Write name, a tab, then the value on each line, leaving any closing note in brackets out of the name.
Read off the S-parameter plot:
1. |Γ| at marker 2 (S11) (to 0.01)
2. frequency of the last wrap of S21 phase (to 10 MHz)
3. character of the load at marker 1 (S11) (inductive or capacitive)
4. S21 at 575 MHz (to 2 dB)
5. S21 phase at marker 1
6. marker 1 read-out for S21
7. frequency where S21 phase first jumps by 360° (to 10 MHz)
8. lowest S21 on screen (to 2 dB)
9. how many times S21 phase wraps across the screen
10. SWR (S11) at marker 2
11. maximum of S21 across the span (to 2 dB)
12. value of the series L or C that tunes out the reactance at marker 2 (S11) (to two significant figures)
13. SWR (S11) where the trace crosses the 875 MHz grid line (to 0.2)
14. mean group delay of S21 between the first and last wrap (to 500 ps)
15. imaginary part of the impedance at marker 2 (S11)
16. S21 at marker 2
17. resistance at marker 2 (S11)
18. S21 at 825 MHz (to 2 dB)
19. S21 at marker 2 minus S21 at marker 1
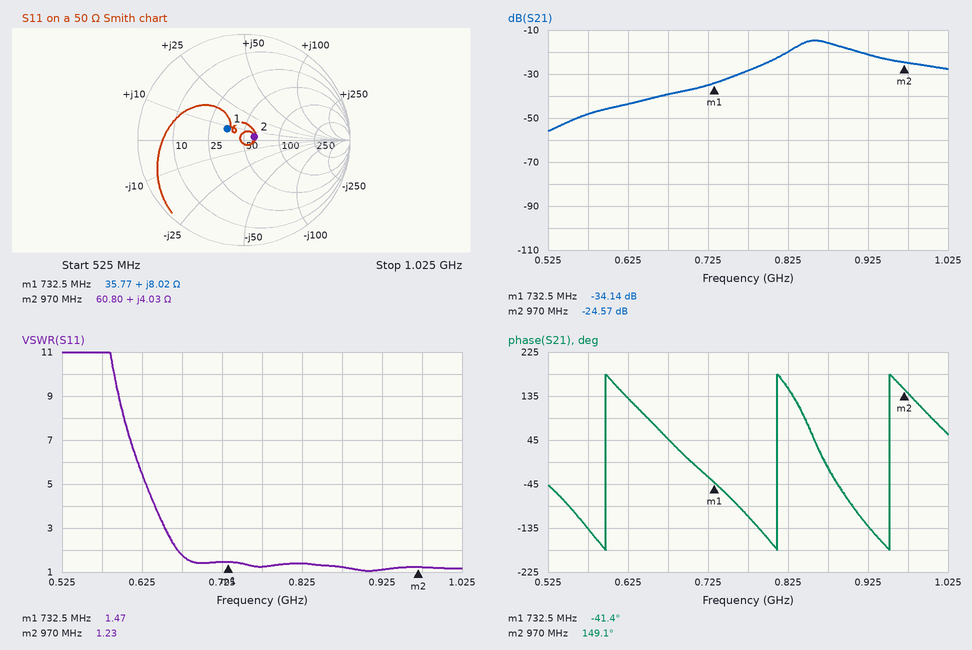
|Γ| at marker 2 (S11)	0.10
frequency of the last wrap of S21 phase	950 MHz
character of the load at marker 1 (S11)	inductive
S21 at 575 MHz	-48 dB
S21 phase at marker 1	-41.4°
marker 1 read-out for S21	-34.14 dB
frequency where S21 phase first jumps by 360°	600 MHz
lowest S21 on screen	-56 dB
how many times S21 phase wraps across the screen	3
SWR (S11) at marker 2	1.23
maximum of S21 across the span	-14 dB
value of the series L or C that tunes out the reactance at marker 2 (S11)	41 pF
SWR (S11) where the trace crosses the 875 MHz grid line	1.2
mean group delay of S21 between the first and last wrap	5.5 ns
imaginary part of the impedance at marker 2	+4.03 Ω
S21 at marker 2	-24.57 dB
resistance at marker 2	60.80 Ω
S21 at 825 MHz	-20 dB
S21 at marker 2 minus S21 at marker 1	9.57 dB
